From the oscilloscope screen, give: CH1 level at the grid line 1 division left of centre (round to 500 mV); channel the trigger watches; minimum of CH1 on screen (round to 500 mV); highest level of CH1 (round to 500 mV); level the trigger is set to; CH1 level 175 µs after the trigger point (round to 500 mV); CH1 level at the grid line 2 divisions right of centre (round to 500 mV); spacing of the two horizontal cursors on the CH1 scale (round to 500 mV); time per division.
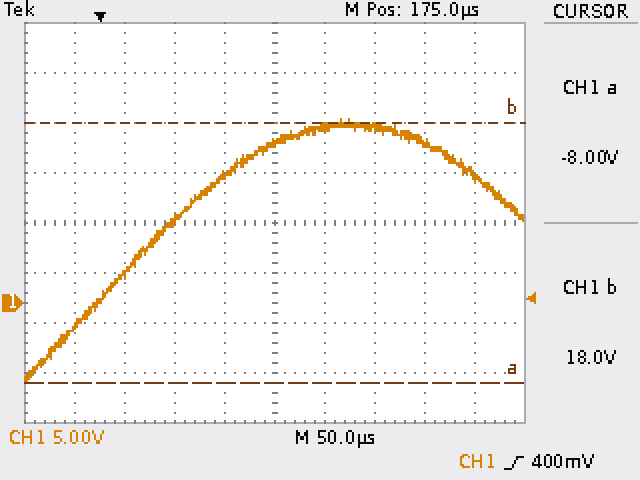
13.0 V
CH1
-8.0 V
18.5 V
400 mV
16.0 V
17.5 V
26.0 V
50 µs
